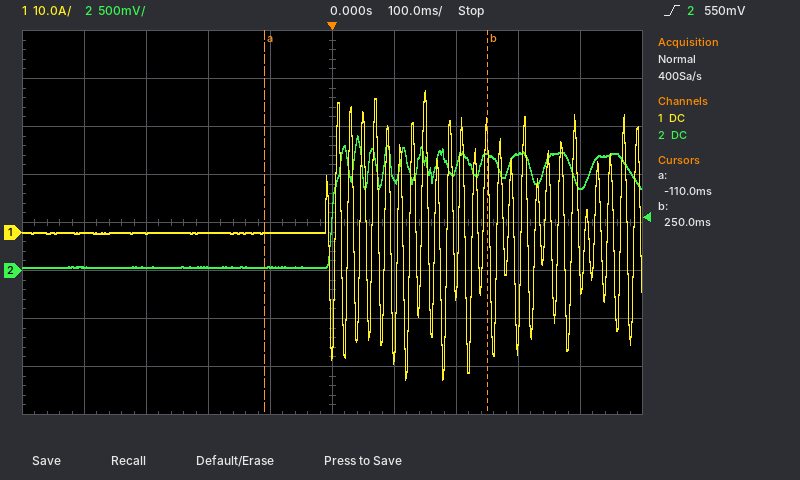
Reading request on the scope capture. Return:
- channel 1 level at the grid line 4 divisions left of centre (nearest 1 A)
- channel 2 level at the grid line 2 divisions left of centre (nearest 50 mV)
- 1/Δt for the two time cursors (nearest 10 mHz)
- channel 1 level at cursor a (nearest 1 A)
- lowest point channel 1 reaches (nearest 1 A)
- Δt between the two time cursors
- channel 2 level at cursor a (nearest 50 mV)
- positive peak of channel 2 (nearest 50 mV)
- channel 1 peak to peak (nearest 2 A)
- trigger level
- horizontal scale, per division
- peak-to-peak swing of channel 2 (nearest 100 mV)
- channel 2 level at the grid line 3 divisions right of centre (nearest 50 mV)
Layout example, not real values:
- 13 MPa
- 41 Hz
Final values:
- 0 A
- 50 mV
- 2.78 Hz
- 0 A
- -31 A
- 360 ms
- 50 mV
- 1.40 V
- 60 A
- 550 mV
- 100 ms
- 1.40 V
- 1.20 V
